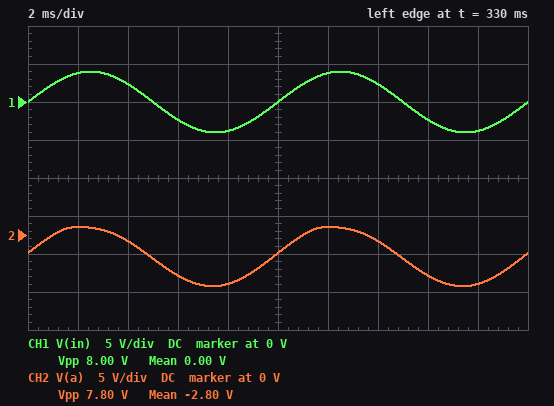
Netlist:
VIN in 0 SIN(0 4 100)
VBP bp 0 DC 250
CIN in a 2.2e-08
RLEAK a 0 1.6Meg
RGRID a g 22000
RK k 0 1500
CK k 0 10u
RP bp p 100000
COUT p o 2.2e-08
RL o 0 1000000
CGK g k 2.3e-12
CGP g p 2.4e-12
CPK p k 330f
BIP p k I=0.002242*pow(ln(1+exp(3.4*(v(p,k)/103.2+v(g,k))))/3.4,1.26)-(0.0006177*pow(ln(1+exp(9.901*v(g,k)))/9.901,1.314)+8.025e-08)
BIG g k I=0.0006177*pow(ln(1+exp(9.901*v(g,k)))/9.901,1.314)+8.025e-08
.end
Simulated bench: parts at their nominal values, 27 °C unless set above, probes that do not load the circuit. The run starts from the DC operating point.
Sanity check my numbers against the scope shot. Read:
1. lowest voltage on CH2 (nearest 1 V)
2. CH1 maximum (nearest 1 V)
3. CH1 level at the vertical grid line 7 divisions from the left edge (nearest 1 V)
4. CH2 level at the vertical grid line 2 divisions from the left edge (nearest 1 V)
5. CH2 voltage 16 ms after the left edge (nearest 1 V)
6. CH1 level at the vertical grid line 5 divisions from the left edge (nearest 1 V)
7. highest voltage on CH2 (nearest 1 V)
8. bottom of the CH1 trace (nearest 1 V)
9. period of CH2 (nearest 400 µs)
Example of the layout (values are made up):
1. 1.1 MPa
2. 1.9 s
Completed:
1. -7 V
2. 4 V
3. 2 V
4. -1 V
5. -5 V
6. 0 V
7. 1 V
8. -4 V
9. 10.0 ms
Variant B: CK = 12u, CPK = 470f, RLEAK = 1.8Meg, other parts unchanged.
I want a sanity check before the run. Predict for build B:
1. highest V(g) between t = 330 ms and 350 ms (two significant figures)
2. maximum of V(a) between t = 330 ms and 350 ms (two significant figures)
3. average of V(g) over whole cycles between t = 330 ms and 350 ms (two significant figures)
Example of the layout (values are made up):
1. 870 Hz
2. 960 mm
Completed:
1. 730 mV
2. 1.0 V
3. -2.9 V
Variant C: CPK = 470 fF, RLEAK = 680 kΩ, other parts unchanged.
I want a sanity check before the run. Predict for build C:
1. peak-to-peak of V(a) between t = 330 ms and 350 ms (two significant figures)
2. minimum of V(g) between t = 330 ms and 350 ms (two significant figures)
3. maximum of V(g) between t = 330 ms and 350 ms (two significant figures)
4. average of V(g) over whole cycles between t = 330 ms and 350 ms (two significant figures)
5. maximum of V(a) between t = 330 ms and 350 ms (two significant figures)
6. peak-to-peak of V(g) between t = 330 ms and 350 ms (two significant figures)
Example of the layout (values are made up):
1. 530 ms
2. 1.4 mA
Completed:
1. 7.5 V
2. -6.1 V
3. 910 mV
4. -2.3 V
5. 1.4 V
6. 7.0 V
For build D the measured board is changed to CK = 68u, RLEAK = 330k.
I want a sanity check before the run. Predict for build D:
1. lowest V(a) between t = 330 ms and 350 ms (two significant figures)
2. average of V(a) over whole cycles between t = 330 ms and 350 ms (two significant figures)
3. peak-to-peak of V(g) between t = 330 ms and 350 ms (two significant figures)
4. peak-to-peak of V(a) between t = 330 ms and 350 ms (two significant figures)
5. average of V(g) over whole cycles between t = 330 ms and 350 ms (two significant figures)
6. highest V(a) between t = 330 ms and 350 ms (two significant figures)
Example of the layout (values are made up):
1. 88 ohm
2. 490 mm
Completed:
1. -5.4 V
2. -1.7 V
3. 6.4 V
4. 7.1 V
5. -1.8 V
6. 1.7 V
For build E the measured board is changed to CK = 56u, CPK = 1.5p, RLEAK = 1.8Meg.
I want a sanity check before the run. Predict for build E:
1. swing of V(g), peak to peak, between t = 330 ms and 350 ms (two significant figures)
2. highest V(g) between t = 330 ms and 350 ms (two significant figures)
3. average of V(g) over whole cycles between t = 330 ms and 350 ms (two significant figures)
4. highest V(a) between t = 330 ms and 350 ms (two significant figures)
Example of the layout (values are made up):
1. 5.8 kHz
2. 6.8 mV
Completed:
1. 7.6 V
2. 730 mV
3. -2.9 V
4. 1.0 V
